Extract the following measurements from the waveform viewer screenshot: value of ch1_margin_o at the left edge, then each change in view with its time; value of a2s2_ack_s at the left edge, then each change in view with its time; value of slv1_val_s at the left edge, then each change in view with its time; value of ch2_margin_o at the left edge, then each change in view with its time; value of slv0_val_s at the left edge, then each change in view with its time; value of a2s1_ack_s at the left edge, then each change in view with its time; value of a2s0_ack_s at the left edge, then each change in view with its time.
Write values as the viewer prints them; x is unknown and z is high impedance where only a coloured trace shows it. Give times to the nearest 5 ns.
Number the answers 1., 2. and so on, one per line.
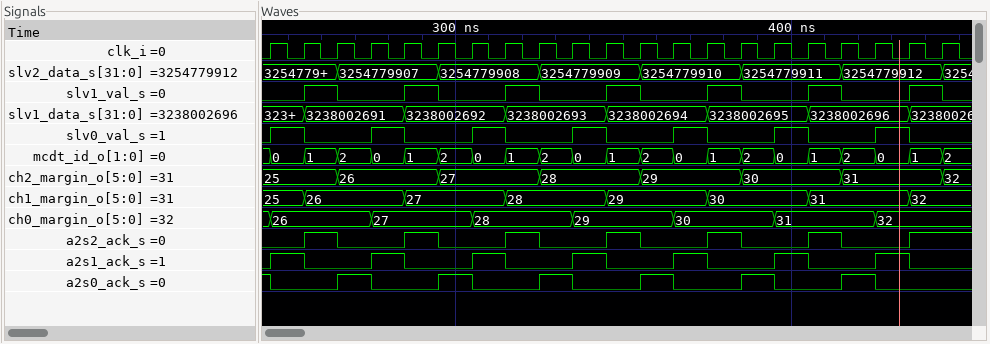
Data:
1. 25, 26 at 255 ns, 27 at 285 ns, 28 at 315 ns, 29 at 345 ns, 30 at 375 ns, 31 at 405 ns, 32 at 435 ns
2. 0, 1 at 255 ns, 0 at 265 ns, 1 at 285 ns, 0 at 295 ns, 1 at 315 ns, 0 at 325 ns, 1 at 345 ns, 0 at 355 ns, 1 at 375 ns, 0 at 385 ns, 1 at 405 ns, 0 at 415 ns, 1 at 435 ns
3. 0, 1 at 255 ns, 0 at 265 ns, 1 at 285 ns, 0 at 295 ns, 1 at 315 ns, 0 at 325 ns, 1 at 345 ns, 0 at 355 ns, 1 at 375 ns, 0 at 385 ns, 1 at 405 ns, 0 at 415 ns, 1 at 435 ns, 0 at 445 ns
4. 25, 26 at 265 ns, 27 at 295 ns, 28 at 325 ns, 29 at 355 ns, 30 at 385 ns, 31 at 415 ns, 32 at 445 ns
5. 0, 1 at 245 ns, 0 at 255 ns, 1 at 275 ns, 0 at 285 ns, 1 at 305 ns, 0 at 315 ns, 1 at 335 ns, 0 at 345 ns, 1 at 365 ns, 0 at 375 ns, 1 at 395 ns, 0 at 405 ns, 1 at 425 ns, 0 at 435 ns
6. 0, 1 at 245 ns, 0 at 255 ns, 1 at 275 ns, 0 at 285 ns, 1 at 305 ns, 0 at 315 ns, 1 at 335 ns, 0 at 345 ns, 1 at 365 ns, 0 at 375 ns, 1 at 395 ns, 0 at 405 ns, 1 at 425 ns, 0 at 435 ns
7. 1, 0 at 245 ns, 1 at 265 ns, 0 at 275 ns, 1 at 295 ns, 0 at 305 ns, 1 at 325 ns, 0 at 335 ns, 1 at 355 ns, 0 at 365 ns, 1 at 385 ns, 0 at 395 ns, 1 at 415 ns, 0 at 425 ns
